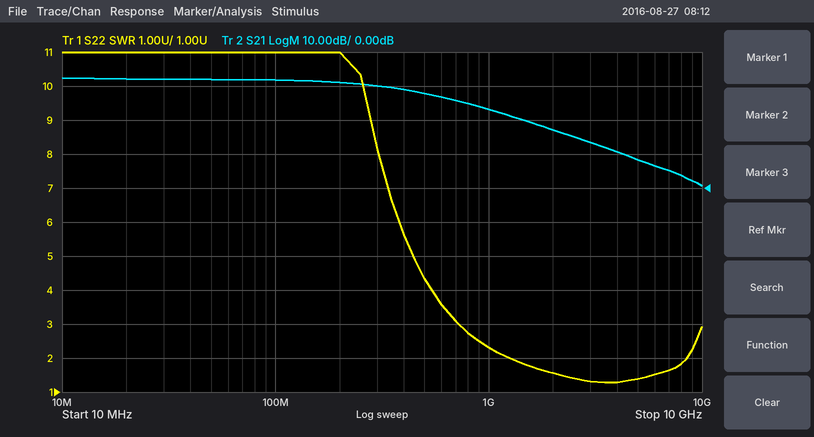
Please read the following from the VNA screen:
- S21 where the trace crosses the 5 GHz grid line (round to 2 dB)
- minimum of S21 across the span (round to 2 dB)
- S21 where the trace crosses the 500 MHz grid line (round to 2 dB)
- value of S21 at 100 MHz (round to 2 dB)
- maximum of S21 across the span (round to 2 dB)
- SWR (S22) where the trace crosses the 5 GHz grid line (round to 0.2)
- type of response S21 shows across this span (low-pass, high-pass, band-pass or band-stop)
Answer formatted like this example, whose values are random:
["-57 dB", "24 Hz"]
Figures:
["8 dB", "0 dB", "28 dB", "32 dB", "32 dB", "1.4", "low-pass"]
